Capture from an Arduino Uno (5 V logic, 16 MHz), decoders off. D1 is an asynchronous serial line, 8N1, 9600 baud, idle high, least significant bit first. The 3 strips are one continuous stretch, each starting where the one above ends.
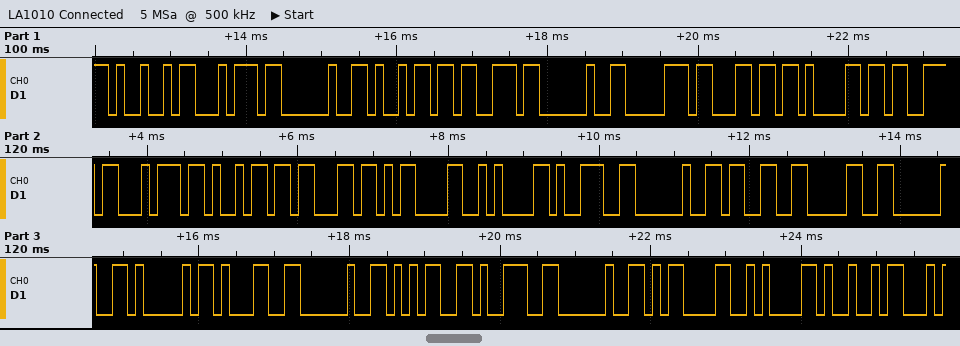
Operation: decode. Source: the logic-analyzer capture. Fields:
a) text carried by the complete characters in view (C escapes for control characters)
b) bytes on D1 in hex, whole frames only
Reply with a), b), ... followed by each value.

a) "It is plastic\r\n9 30 A1 59 \r\nI"
b) 49 74 20 69 73 20 70 6C 61 73 74 69 63 0D 0A 39 20 33 30 20 41 31 20 35 39 20 0D 0A 49
